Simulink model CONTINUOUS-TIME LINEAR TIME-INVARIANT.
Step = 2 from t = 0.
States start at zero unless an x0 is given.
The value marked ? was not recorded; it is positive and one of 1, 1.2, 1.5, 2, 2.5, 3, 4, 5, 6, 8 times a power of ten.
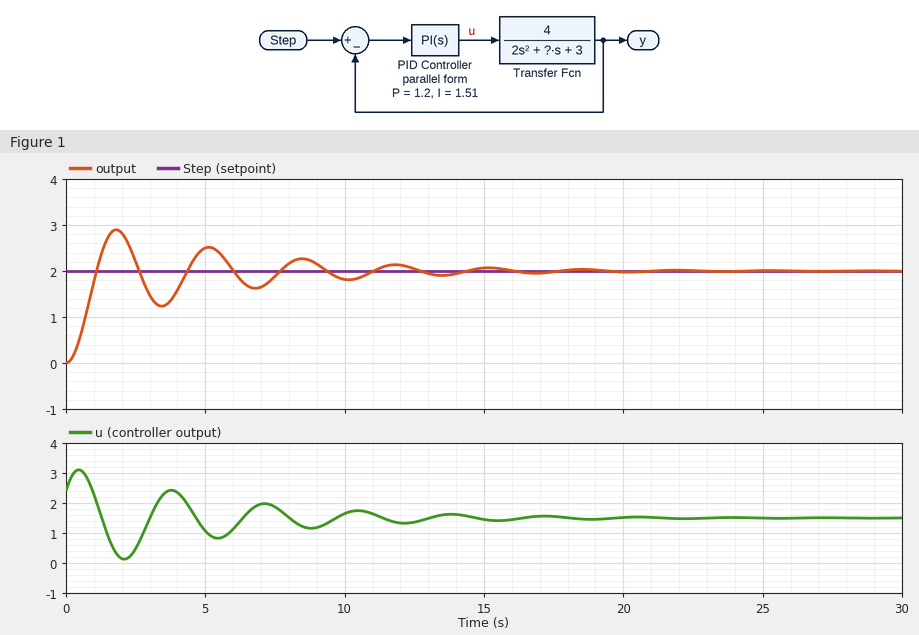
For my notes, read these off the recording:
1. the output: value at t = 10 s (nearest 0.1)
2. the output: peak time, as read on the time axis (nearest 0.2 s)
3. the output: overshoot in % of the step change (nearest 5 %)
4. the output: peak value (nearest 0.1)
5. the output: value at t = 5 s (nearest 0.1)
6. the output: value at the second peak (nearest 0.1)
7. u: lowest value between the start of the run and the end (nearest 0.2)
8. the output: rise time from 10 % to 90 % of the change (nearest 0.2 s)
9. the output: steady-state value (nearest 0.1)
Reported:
1.8
1.8 s
45 %
2.9
2.5
2.5
0.2
0.8 s
2.0
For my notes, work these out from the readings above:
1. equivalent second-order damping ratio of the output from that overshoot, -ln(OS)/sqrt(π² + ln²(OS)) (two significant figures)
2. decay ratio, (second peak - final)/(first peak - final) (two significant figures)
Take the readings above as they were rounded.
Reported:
0.25
0.56
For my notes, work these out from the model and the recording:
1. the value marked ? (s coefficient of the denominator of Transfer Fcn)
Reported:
2.5
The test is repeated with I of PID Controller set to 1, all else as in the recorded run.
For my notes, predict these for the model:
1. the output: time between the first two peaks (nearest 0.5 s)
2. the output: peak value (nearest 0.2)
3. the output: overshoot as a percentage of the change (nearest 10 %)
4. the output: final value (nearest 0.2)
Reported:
3.5 s
2.6
30 %
2.0
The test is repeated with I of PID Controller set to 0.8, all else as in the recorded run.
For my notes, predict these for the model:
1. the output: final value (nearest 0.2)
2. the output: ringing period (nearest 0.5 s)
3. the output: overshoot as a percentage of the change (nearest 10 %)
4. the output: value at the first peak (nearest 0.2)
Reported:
2.0
3.5 s
20 %
2.4
